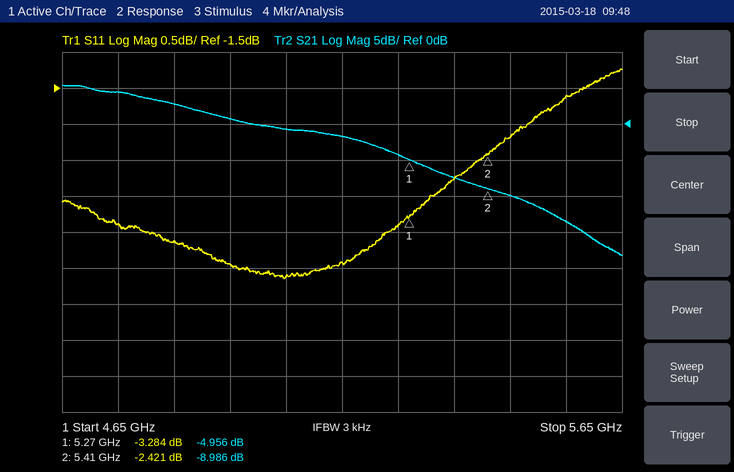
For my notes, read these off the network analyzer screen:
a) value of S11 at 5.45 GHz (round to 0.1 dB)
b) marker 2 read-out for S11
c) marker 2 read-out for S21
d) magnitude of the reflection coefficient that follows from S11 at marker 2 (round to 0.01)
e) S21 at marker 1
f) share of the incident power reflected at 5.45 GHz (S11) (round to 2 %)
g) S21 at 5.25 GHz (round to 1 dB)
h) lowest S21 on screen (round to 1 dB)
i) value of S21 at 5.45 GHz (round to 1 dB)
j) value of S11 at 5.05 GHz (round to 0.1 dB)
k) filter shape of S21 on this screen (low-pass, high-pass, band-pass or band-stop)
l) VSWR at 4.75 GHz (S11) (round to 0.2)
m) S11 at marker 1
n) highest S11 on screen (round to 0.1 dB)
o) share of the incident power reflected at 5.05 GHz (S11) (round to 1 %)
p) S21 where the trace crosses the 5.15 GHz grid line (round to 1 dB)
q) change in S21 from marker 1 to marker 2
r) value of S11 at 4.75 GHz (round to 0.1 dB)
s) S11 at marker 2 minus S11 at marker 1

-2.2 dB
-2.421 dB
-8.986 dB
0.76
-4.956 dB
60 %
-4 dB
-18 dB
-10 dB
-4.1 dB
low-pass
5.2
-3.284 dB
-1.2 dB
39 %
-2 dB
-4.030 dB
-3.4 dB
0.863 dB
